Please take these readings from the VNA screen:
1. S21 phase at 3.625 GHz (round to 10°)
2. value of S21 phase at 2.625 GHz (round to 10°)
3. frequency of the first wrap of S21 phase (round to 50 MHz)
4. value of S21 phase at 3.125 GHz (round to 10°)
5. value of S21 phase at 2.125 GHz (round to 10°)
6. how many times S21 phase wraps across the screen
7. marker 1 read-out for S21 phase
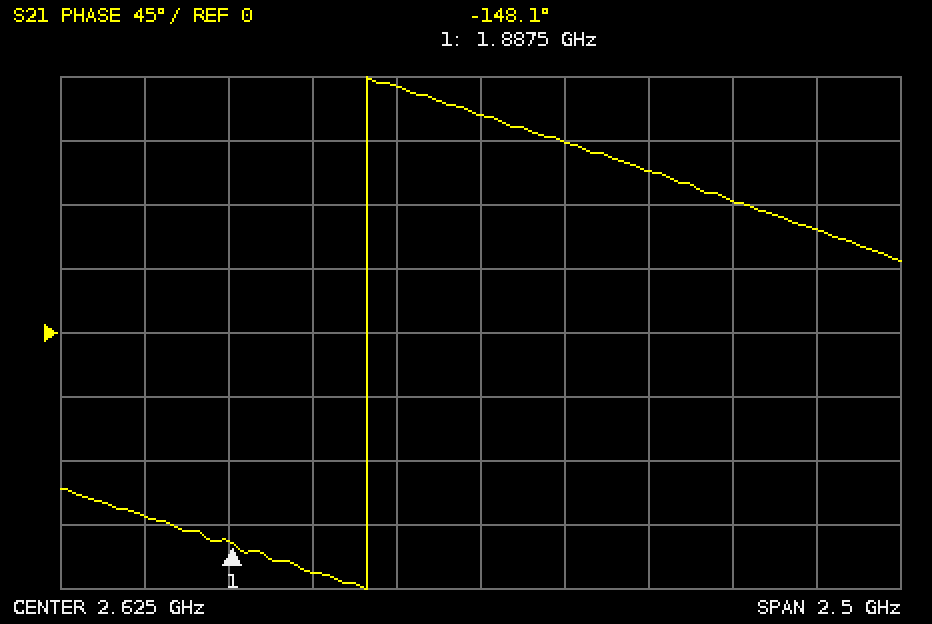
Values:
70°
150°
2.30 GHz
110°
-170°
1
-148.1°
